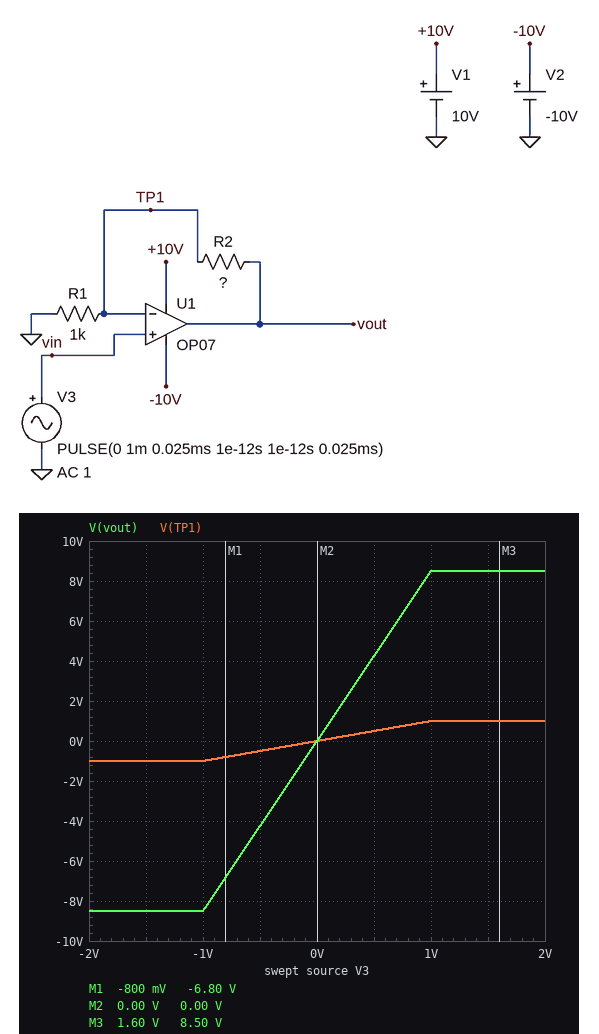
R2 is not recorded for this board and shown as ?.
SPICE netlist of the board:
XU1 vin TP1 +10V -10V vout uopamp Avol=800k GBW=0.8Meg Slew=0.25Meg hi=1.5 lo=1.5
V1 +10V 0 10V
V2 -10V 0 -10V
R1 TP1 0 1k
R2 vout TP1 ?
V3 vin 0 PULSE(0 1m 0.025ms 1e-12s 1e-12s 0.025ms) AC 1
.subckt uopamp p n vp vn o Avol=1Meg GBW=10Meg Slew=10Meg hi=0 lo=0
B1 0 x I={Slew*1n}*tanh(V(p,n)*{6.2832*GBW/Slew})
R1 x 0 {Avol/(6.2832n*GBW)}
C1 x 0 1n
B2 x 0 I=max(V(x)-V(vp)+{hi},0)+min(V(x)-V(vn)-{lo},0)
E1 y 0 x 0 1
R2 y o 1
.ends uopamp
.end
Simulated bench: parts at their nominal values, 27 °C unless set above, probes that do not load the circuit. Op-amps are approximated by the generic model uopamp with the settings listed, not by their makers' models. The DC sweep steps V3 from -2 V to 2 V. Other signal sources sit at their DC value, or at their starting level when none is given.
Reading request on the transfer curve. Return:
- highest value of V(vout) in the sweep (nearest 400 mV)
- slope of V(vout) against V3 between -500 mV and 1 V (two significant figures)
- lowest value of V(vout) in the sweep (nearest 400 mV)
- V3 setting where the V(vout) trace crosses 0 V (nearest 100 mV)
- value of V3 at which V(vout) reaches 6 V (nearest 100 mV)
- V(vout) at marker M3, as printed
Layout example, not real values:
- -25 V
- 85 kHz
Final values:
- 8.4 V
- 8.5 V/V
- -8.4 V
- 0 V
- 700 mV
- 8.50 V
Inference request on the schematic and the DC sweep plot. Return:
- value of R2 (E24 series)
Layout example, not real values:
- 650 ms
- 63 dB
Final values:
- 7.5 kΩ
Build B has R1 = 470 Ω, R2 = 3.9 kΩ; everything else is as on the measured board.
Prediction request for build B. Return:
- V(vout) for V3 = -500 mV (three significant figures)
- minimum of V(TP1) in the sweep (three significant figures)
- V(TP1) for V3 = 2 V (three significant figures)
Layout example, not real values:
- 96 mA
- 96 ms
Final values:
- -4.65 V
- -914 mV
- 914 mV
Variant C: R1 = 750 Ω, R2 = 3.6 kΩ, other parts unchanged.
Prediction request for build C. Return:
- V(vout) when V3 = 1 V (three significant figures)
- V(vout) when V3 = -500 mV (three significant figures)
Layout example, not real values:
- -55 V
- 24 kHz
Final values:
- 5.80 V
- -2.90 V
